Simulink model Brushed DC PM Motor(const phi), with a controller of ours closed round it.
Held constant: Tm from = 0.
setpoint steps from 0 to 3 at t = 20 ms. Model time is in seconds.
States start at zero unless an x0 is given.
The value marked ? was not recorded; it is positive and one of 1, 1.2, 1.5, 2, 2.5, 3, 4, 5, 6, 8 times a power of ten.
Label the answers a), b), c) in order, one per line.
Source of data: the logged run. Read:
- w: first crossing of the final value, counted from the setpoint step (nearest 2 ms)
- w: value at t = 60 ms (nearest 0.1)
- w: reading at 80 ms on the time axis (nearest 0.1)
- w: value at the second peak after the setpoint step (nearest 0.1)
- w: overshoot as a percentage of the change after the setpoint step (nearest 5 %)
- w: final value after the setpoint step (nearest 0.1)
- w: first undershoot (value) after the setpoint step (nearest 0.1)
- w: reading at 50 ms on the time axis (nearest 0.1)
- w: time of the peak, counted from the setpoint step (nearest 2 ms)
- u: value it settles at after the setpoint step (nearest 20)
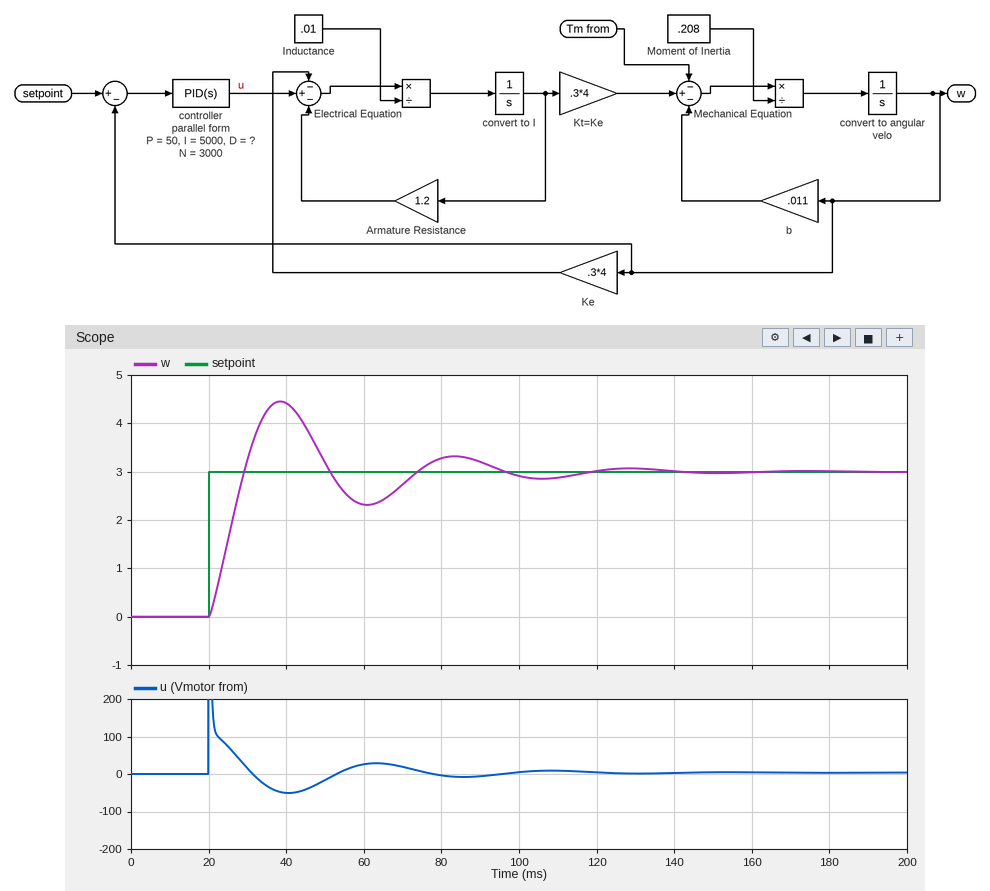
a) 10 ms
b) 2.3
c) 3.3
d) 3.3
e) 50 %
f) 3.0
g) 2.3
h) 3.2
i) 18 ms
j) 0
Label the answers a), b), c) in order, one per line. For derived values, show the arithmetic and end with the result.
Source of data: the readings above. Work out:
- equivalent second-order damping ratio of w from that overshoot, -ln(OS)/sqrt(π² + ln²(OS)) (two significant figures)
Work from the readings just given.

a) ln(0.5) = -0.693; 0.693 / sqrt(9.870 + 0.480) = 0.22
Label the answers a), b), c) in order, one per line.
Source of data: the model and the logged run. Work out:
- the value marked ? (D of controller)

a) 0.15
